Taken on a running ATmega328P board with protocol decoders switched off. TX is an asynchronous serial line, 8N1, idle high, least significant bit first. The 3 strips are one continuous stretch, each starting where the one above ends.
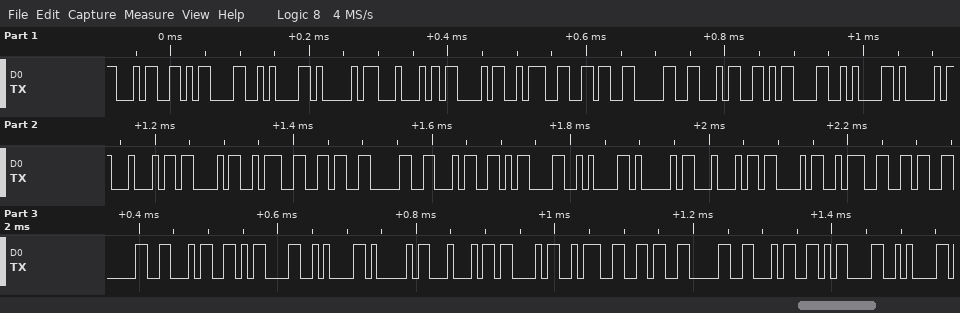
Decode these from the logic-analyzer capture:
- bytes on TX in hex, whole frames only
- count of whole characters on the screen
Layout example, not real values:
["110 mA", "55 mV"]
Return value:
["34 0D 0A 41 44 43 3A 36 30 34 0D 0A 41 44 43 3A 36 30 34 0D 0A 41 44 43 3A 36 30 34 0D 0A 41 44 43 3A 36 30 34 0D 0A", "39"]
